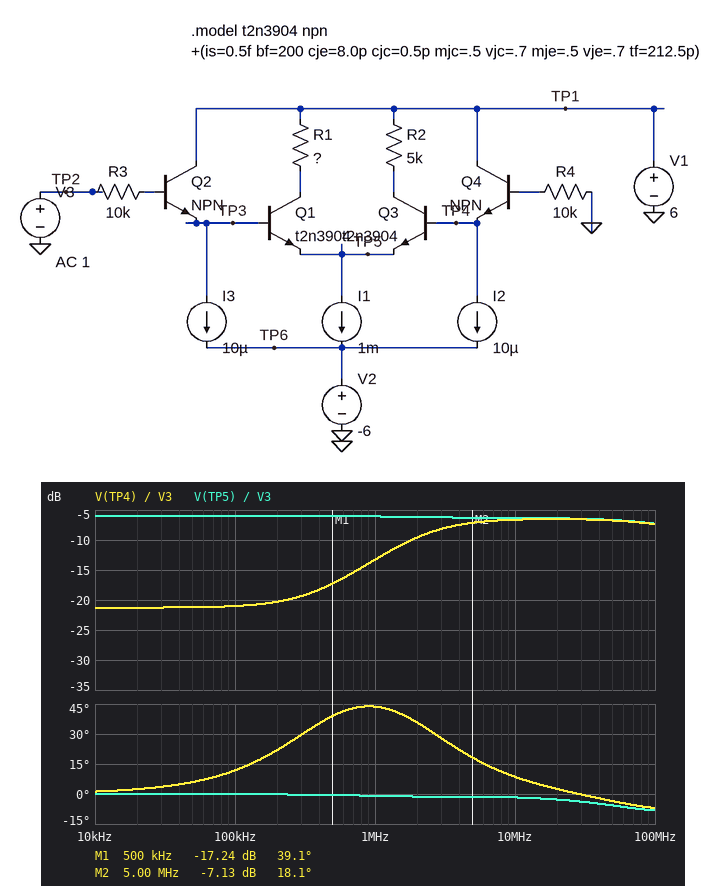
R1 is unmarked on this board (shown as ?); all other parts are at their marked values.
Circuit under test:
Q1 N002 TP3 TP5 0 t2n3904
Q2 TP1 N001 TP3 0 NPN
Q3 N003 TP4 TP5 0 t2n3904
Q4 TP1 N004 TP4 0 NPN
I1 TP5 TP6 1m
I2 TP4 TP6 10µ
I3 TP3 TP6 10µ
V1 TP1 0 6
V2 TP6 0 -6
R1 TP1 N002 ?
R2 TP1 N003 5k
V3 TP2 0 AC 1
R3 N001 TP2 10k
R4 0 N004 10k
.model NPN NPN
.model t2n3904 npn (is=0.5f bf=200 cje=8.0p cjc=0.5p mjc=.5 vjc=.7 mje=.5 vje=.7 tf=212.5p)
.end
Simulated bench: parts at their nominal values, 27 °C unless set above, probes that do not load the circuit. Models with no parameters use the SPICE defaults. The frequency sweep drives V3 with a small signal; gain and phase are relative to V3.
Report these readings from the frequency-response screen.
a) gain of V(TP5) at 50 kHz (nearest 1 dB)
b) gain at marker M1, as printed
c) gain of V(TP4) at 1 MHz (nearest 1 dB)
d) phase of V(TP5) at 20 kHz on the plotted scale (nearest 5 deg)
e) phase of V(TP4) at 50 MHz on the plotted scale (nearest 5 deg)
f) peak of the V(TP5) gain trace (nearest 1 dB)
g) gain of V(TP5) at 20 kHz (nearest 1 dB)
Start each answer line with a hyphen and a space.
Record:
- -6 dB
- -17.24 dB
- -13 dB
- 0 deg
- -5 deg
- -6 dB
- -6 dB
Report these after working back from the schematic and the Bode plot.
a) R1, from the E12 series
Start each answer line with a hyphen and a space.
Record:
- 5.6 kΩ
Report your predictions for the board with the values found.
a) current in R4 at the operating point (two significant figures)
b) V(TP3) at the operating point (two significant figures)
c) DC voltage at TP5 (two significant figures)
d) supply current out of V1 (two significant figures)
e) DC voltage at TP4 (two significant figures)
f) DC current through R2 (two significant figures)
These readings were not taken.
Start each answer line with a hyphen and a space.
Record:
- 120 nA
- -660 mV
- -1.4 V
- 1.0 mA
- -660 mV
- 500 µA
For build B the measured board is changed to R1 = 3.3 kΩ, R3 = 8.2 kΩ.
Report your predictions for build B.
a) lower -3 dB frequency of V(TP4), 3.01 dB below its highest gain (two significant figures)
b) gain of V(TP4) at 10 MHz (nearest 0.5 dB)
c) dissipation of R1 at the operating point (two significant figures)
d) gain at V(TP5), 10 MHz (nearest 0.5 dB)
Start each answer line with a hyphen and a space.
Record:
- 2.3 MHz
- -5.5 dB
- 820 µW
- -5.0 dB
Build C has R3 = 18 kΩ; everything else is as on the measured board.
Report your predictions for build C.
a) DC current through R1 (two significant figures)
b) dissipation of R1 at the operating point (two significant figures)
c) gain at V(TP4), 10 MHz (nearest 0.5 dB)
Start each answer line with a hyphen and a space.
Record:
- 490 µA
- 1.3 mW
- -7.0 dB
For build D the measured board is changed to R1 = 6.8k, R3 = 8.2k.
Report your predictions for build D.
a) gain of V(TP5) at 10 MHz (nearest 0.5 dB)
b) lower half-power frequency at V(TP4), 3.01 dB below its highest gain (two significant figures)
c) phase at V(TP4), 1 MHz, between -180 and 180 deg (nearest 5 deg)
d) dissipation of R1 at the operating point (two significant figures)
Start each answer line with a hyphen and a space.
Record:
- -7.0 dB
- 1.9 MHz
- 40 deg
- 1.7 mW
